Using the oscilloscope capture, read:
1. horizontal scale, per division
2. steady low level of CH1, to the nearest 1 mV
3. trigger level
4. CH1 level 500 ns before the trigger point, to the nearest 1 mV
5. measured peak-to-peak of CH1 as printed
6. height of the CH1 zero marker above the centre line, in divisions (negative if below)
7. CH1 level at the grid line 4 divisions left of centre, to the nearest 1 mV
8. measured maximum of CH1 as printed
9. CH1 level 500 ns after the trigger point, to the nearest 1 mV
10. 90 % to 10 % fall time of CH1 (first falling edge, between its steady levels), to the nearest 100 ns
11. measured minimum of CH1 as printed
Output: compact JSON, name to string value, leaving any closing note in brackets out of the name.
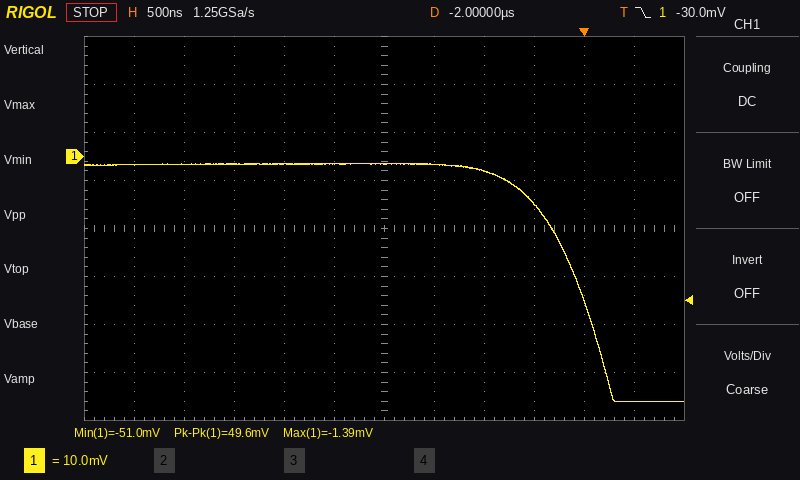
{"horizontal scale, per division": "500 ns", "steady low level of CH1, to the nearest 1 mV": "-51 mV", "trigger level": "-30.0 mV", "CH1 level 500 ns before the trigger point, to the nearest 1 mV": "-10 mV", "measured peak-to-peak of CH1 as printed": "49.6 mV", "height of the CH1 zero marker above the centre line, in divisions": "+1.5 div", "CH1 level at the grid line 4 divisions left of centre, to the nearest 1 mV": "-2 mV", "measured maximum of CH1 as printed": "-1.39 mV", "CH1 level 500 ns after the trigger point, to the nearest 1 mV": "-51 mV", "90 % to 10 % fall time of CH1 (first falling edge, between its steady levels), to the nearest 100 ns": "900 ns", "measured minimum of CH1 as printed": "-51.0 mV"}
